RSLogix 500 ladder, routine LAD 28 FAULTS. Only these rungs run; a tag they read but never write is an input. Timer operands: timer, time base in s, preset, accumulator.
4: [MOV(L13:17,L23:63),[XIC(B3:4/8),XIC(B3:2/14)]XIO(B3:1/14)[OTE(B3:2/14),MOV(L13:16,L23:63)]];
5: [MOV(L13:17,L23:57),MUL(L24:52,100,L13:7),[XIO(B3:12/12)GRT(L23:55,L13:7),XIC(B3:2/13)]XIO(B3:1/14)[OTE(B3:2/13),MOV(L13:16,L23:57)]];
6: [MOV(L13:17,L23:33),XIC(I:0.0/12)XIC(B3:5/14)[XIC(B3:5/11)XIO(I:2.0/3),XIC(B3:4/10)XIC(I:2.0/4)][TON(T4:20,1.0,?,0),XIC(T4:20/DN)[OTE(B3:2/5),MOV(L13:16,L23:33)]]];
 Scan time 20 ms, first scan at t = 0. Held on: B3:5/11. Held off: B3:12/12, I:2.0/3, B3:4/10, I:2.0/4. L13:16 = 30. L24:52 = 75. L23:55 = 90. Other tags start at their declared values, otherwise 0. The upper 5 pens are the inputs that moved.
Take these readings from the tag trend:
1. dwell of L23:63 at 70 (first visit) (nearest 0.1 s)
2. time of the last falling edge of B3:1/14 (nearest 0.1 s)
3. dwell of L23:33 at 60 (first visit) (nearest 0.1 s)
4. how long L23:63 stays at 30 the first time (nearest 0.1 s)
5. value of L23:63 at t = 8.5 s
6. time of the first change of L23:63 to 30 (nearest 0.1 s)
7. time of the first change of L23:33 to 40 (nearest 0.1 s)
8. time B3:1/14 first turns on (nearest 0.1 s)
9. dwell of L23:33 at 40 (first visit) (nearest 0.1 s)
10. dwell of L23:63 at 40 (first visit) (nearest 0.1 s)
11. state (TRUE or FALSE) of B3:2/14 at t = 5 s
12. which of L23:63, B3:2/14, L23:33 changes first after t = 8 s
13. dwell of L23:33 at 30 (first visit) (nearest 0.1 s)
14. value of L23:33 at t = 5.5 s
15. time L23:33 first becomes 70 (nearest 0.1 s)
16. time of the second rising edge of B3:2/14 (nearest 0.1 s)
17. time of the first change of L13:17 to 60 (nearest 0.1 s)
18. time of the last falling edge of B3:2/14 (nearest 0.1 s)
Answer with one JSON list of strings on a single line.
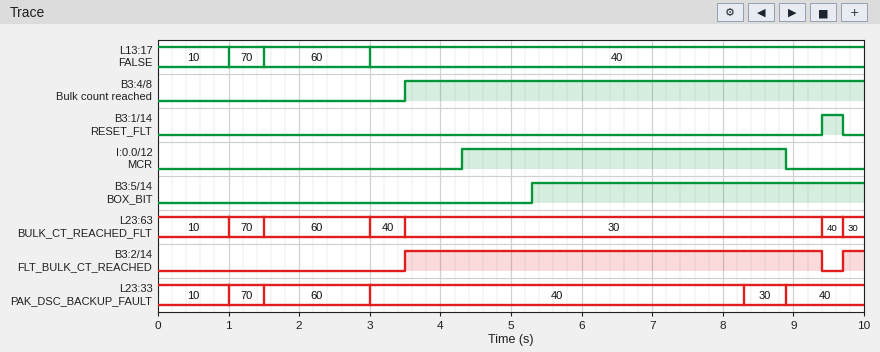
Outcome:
["0.5 s", "9.7 s", "1.5 s", "5.9 s", "30", "3.5 s", "3.0 s", "9.4 s", "5.3 s", "0.5 s", "TRUE", "L23:33", "0.6 s", "40", "1.0 s", "9.7 s", "1.5 s", "9.4 s"]
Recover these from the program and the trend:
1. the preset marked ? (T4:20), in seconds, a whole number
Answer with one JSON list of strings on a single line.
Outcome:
["3 s"]
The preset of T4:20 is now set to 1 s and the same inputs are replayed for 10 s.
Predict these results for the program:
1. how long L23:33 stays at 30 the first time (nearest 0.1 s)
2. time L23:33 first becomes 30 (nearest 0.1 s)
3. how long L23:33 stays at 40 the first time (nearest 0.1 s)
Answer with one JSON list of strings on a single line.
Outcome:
["2.6 s", "6.3 s", "3.3 s"]
